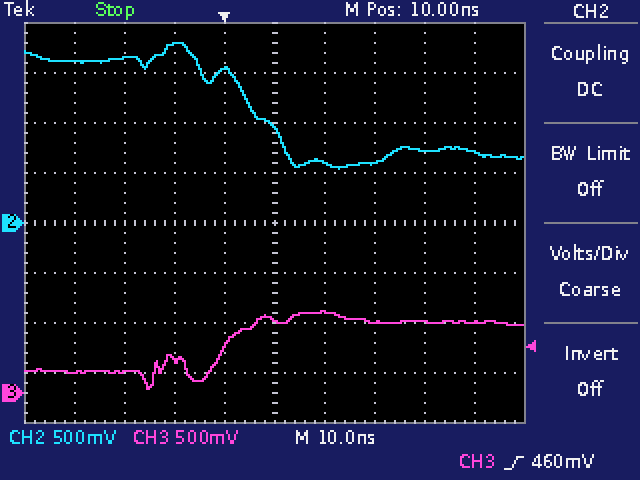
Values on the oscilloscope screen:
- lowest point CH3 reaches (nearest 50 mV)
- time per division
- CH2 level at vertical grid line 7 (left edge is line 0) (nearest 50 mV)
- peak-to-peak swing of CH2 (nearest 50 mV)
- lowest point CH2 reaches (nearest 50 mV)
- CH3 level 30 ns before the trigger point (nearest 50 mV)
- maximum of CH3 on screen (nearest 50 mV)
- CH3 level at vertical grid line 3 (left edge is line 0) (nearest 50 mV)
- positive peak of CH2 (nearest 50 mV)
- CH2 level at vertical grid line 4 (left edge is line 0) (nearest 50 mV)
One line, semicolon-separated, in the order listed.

50 mV; 10 ns; 600 mV; 1.25 V; 550 mV; 200 mV; 800 mV; 350 mV; 1.80 V; 1.55 V
